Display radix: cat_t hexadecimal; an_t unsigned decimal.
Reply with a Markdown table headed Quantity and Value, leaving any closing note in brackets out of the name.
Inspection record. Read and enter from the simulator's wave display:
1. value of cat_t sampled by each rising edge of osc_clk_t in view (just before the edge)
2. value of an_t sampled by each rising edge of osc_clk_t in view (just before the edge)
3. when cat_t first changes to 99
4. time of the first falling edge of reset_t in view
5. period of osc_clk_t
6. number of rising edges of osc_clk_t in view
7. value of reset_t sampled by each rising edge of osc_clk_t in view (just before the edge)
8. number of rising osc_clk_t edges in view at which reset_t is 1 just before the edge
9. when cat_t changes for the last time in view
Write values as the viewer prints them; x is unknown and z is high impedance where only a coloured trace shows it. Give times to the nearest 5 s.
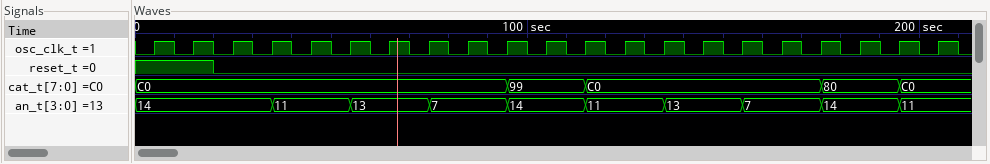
| Quantity | Value |
|---|---|
| value of cat_t sampled by each rising edge of osc_clk_t in view | C0, C0, C0, C0, C0, C0, C0, C0, C0, C0, 99, 99, C0, C0, C0, C0, C0, C0, 80, 80, C0 |
| value of an_t sampled by each rising edge of osc_clk_t in view | 14, 14, 14, 14, 11, 11, 13, 13, 7, 7, 14, 14, 11, 11, 13, 13, 7, 7, 14, 14, 11 |
| when cat_t first changes to 99 | 95 s |
| time of the first falling edge of reset_t in view | 20 s |
| period of osc_clk_t | 10 s |
| number of rising edges of osc_clk_t in view | 21 |
| value of reset_t sampled by each rising edge of osc_clk_t in view | 1 1 0 0 0 0 0 0 0 0 0 0 0 0 0 0 0 0 0 0 0 |
| number of rising osc_clk_t edges in view at which reset_t is 1 just before the edge | 2 |
| when cat_t changes for the last time in view | 195 s |
